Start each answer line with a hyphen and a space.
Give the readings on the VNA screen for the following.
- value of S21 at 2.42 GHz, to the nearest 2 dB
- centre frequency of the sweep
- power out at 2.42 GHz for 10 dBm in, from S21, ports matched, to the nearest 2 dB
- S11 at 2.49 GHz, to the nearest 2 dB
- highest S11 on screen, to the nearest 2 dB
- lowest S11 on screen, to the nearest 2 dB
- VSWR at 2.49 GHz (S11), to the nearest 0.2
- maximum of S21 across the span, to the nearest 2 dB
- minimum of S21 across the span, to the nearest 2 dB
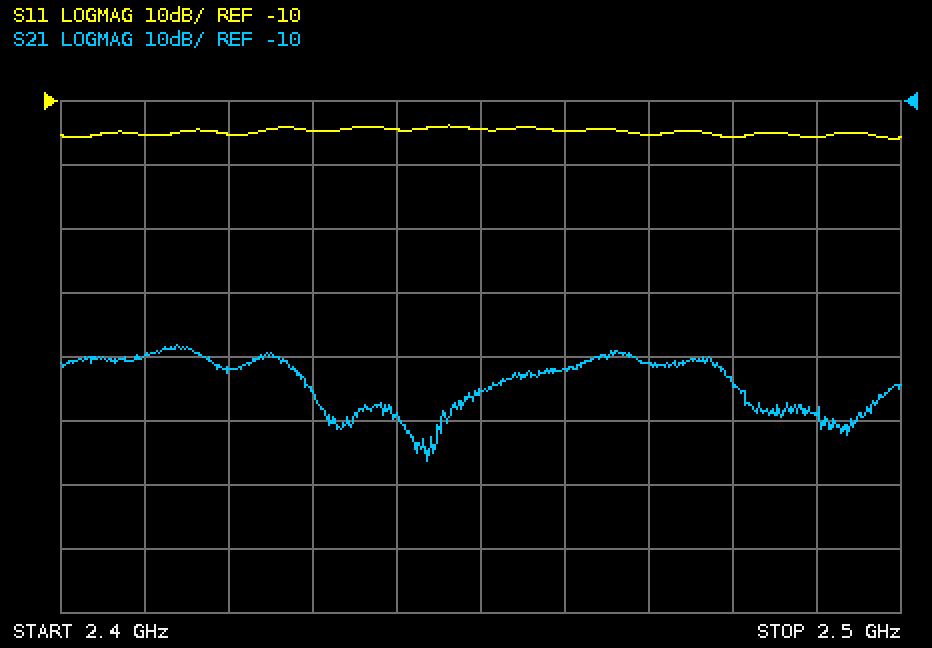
- -52 dB
- 2.45 GHz
- -42 dBm
- -16 dB
- -14 dB
- -16 dB
- 1.4
- -48 dB
- -66 dB
